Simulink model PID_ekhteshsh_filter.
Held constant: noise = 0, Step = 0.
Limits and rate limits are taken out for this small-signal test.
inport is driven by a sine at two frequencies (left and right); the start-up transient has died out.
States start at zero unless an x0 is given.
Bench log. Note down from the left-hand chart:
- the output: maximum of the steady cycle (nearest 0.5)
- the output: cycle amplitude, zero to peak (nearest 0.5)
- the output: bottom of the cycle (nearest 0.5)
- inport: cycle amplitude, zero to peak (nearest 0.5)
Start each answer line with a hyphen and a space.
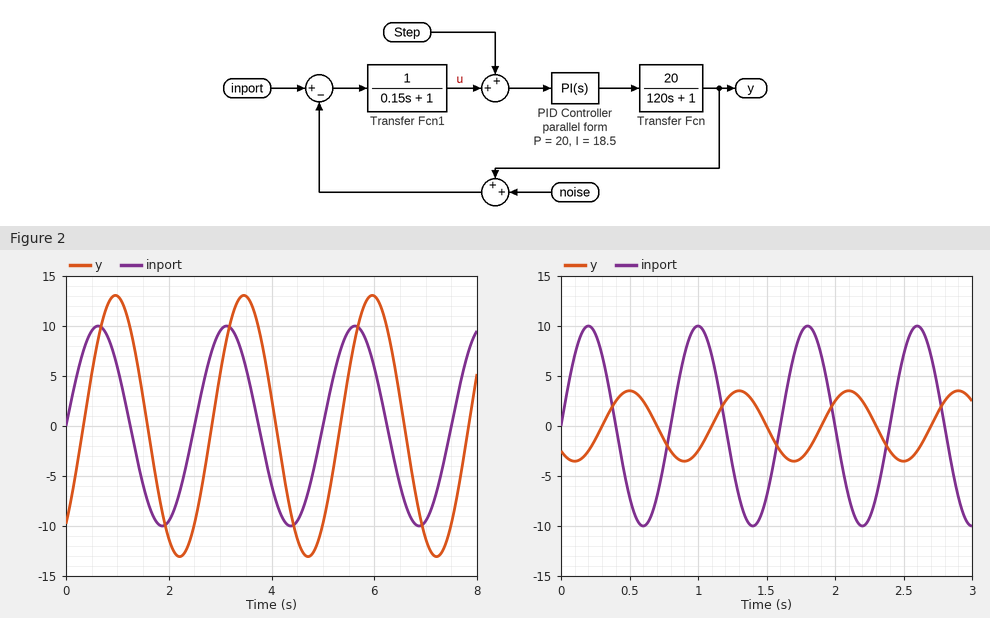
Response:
- 13.0
- 13.0
- -13.0
- 10.0
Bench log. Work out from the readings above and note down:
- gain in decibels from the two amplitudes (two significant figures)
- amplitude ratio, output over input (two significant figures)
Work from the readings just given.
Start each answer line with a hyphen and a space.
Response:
- 2.3 dB
- 1.3
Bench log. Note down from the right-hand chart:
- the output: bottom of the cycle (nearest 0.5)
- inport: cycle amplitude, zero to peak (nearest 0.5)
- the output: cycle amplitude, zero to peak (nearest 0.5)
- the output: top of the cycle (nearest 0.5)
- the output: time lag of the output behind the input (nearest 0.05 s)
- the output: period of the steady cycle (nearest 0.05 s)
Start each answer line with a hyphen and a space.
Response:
- -3.5
- 10.0
- 3.5
- 3.5
- 0.30 s
- 0.80 s
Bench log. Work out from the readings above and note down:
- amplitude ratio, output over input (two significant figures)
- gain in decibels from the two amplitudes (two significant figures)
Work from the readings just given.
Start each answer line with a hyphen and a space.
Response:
- 0.35
- -9.1 dB
